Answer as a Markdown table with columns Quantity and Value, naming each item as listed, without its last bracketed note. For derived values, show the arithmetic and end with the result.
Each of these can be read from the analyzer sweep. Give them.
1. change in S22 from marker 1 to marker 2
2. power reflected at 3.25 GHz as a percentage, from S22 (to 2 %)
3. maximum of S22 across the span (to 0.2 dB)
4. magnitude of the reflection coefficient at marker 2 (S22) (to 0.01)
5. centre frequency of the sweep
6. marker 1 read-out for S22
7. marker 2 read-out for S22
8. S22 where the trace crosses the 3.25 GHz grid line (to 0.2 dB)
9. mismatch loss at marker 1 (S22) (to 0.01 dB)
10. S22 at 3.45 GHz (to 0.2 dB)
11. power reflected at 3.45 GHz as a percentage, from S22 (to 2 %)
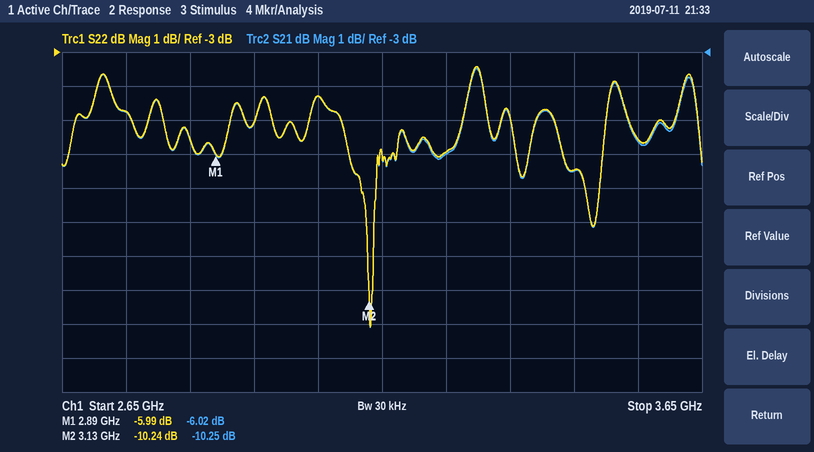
| Quantity | Value |
|---|---|
| change in S22 from marker 1 to marker 2 | -10.24 − (-5.99) = -4.25 dB |
| power reflected at 3.25 GHz as a percentage, from S22 | 10^(-6/10) ≈ 25.1 %, so 26 % to the nearest 2 % |
| maximum of S22 across the span | -3.4 dB |
| magnitude of the reflection coefficient at marker 2 (S22) | 10^(-10.24/20) ≈ 0.31 |
| centre frequency of the sweep | 3.15 GHz |
| marker 1 read-out for S22 | -5.99 dB |
| marker 2 read-out for S22 | -10.24 dB |
| S22 where the trace crosses the 3.25 GHz grid line | -6.0 dB |
| mismatch loss at marker 1 (S22) | −10 log10(1 − 10^(-5.99/10)) ≈ 1.26 dB |
| S22 at 3.45 GHz | -6.4 dB |
| power reflected at 3.45 GHz as a percentage, from S22 | 10^(-6.4/10) ≈ 22.9 %, so 22 % to the nearest 2 % |
